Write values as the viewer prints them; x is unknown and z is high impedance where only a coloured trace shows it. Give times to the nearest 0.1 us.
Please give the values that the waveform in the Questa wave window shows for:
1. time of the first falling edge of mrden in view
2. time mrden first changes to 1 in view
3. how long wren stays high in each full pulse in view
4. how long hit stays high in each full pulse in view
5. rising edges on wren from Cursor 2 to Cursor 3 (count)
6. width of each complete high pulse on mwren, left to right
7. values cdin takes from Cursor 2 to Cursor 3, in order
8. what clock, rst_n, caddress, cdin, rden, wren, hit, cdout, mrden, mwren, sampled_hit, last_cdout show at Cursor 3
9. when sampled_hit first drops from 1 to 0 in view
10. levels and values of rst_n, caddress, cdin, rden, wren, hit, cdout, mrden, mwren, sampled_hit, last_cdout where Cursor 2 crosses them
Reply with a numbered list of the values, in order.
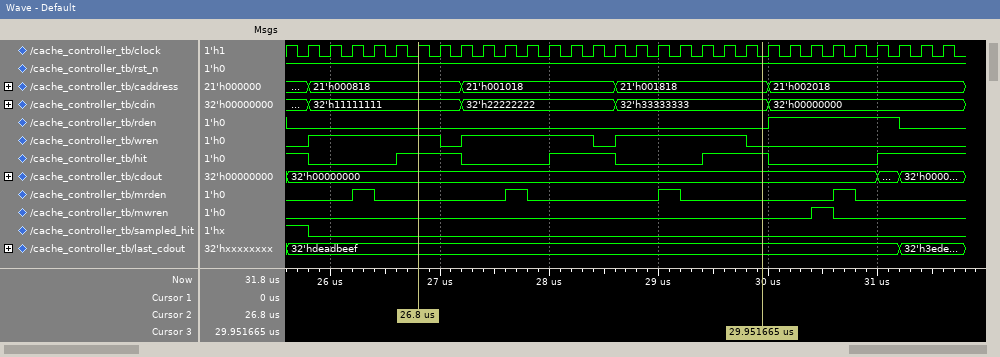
1. 26.4 us
2. 26.2 us
3. 1.2 us, 1.2 us, 1.2 us
4. 0.6 us, 0.6 us, 0.6 us
5. 2
6. 0.2 us
7. 32'h11111111, 32'h22222222, 32'h33333333
8. clock=0, rst_n=1, caddress=21'h001818, cdin=32'h33333333, rden=0, wren=0, hit=1, cdout=32'h00000000, mrden=0, mwren=0, sampled_hit=0, last_cdout=32'hdeadbeef
9. 25.8 us
10. rst_n=1, caddress=21'h000818, cdin=32'h11111111, rden=0, wren=1, hit=1, cdout=32'h00000000, mrden=0, mwren=0, sampled_hit=0, last_cdout=32'hdeadbeef
